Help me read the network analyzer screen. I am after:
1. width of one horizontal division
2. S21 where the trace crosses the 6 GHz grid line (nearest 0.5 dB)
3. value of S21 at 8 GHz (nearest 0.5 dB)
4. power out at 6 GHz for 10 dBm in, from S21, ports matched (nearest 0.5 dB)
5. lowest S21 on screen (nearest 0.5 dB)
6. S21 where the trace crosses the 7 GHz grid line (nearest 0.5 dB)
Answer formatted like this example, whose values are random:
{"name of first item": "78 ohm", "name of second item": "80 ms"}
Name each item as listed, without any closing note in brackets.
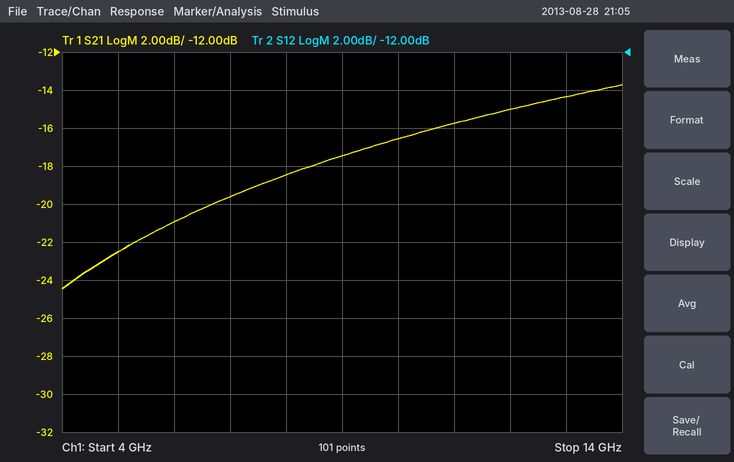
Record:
{"width of one horizontal division": "1 GHz", "S21 where the trace crosses the 6 GHz grid line": "-21.0 dB", "value of S21 at 8 GHz": "-18.5 dB", "power out at 6 GHz for 10 dBm in, from S21, ports matched": "-11.0 dBm", "lowest S21 on screen": "-24.5 dB", "S21 where the trace crosses the 7 GHz grid line": "-19.5 dB"}
